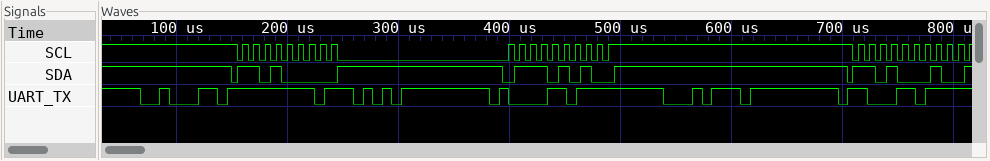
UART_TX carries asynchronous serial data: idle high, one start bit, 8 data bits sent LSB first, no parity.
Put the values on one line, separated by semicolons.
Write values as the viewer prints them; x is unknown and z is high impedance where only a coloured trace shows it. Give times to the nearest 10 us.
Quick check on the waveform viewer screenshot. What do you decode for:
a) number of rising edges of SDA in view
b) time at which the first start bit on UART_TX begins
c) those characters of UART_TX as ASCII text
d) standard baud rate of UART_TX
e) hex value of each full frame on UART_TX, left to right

11; 70 us; "bWatc"; 115200 baud; 62, 57, 61, 74, 63
